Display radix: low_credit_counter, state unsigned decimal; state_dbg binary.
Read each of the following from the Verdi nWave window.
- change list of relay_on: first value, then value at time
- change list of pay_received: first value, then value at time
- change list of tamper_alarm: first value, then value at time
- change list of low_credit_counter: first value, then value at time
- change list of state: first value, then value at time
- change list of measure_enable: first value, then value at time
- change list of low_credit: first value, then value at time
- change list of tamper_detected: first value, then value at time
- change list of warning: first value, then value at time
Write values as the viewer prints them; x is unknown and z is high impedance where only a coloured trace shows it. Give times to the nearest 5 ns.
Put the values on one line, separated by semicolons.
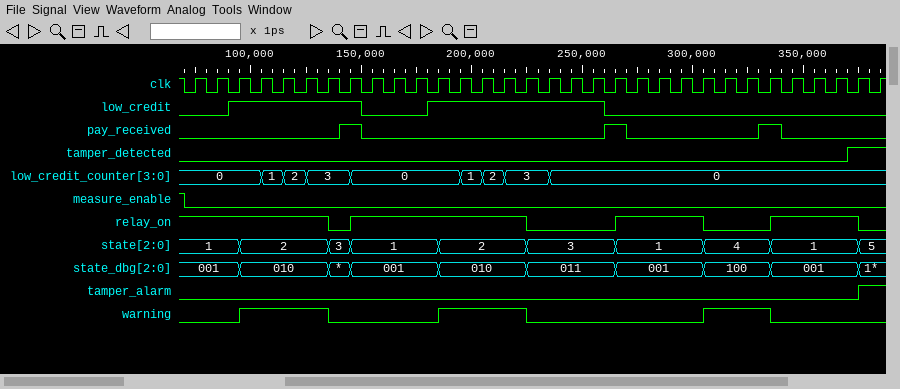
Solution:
1, 0 at 135 ns, 1 at 145 ns, 0 at 225 ns, 1 at 265 ns, 0 at 305 ns, 1 at 335 ns, 0 at 375 ns; 0, 1 at 140 ns, 0 at 150 ns, 1 at 260 ns, 0 at 270 ns, 1 at 330 ns, 0 at 340 ns; 0, 1 at 375 ns; 0, 1 at 105 ns, 2 at 115 ns, 3 at 125 ns, 0 at 145 ns, 1 at 195 ns, 2 at 205 ns, 3 at 215 ns, 0 at 235 ns; 1, 2 at 95 ns, 3 at 135 ns, 1 at 145 ns, 2 at 185 ns, 3 at 225 ns, 1 at 265 ns, 4 at 305 ns, 1 at 335 ns, 5 at 375 ns; 1, 0 at 70 ns; 0, 1 at 90 ns, 0 at 150 ns, 1 at 180 ns, 0 at 260 ns; 0, 1 at 370 ns; 0, 1 at 95 ns, 0 at 135 ns, 1 at 185 ns, 0 at 225 ns, 1 at 305 ns, 0 at 335 ns
